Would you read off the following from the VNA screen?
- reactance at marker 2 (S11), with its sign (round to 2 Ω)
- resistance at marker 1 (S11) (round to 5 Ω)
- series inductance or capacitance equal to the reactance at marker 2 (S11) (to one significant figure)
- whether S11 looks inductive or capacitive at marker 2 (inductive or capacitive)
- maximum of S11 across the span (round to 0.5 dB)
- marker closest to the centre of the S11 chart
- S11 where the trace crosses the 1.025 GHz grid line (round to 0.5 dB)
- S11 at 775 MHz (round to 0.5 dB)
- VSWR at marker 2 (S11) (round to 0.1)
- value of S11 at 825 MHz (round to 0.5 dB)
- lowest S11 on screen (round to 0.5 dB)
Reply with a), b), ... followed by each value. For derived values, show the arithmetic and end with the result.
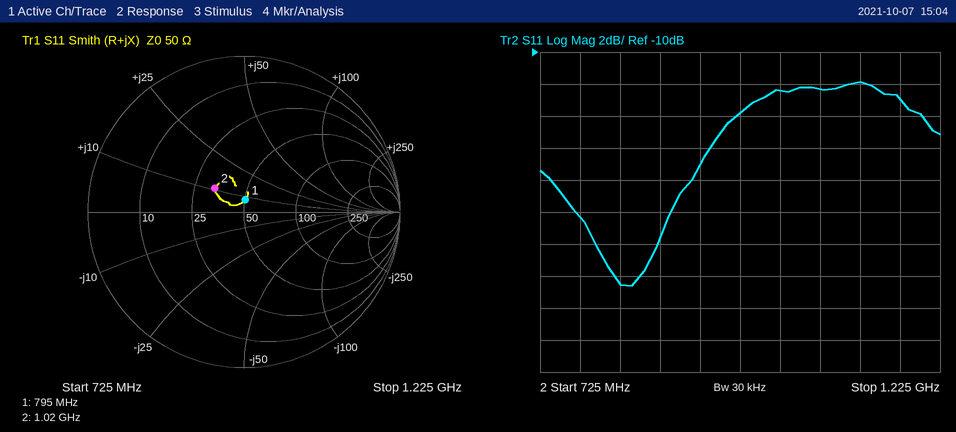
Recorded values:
a) +10 Ω
b) 50 Ω
c) L = 10 Ω/(2π × 1.02 GHz) ≈ 2 nH
d) inductive
e) -12.0 dB
f) marker 1
g) -12.5 dB
h) -20.5 dB
i) 1.6
j) -24.5 dB
k) -24.5 dB
